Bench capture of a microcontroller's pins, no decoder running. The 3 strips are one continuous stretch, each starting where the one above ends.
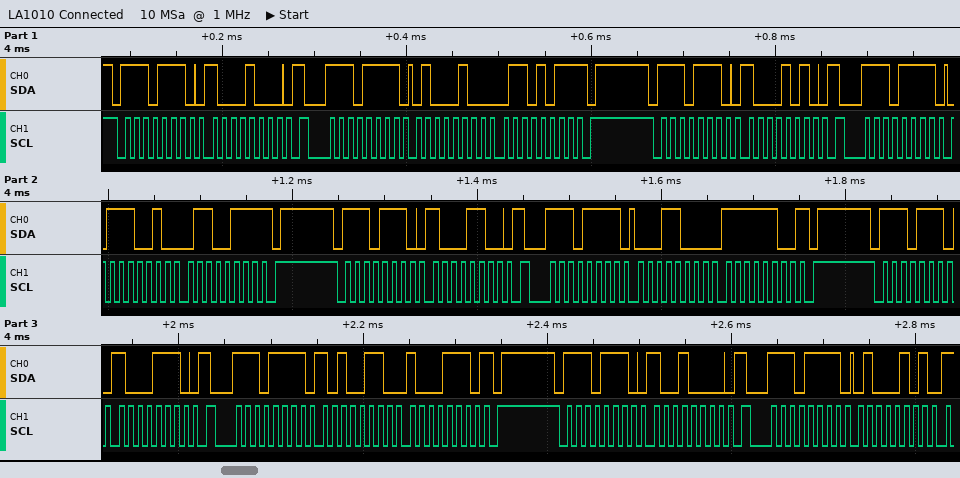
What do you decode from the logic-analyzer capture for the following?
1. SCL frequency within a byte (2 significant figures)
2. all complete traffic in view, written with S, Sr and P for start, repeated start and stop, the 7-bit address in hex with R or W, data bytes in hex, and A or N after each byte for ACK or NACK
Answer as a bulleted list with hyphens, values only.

- 100 kHz
- S 77W A 88 A Sr 77R A 44 A 6B N P S 77W A 8A A Sr 77R A 72 A 67 N P S 77W A 8C A Sr 77R A 18 A FC N P S 77W A 8E A Sr 77R A A6 A 8E N P S 77W A 90 A Sr 77R A 45 A
